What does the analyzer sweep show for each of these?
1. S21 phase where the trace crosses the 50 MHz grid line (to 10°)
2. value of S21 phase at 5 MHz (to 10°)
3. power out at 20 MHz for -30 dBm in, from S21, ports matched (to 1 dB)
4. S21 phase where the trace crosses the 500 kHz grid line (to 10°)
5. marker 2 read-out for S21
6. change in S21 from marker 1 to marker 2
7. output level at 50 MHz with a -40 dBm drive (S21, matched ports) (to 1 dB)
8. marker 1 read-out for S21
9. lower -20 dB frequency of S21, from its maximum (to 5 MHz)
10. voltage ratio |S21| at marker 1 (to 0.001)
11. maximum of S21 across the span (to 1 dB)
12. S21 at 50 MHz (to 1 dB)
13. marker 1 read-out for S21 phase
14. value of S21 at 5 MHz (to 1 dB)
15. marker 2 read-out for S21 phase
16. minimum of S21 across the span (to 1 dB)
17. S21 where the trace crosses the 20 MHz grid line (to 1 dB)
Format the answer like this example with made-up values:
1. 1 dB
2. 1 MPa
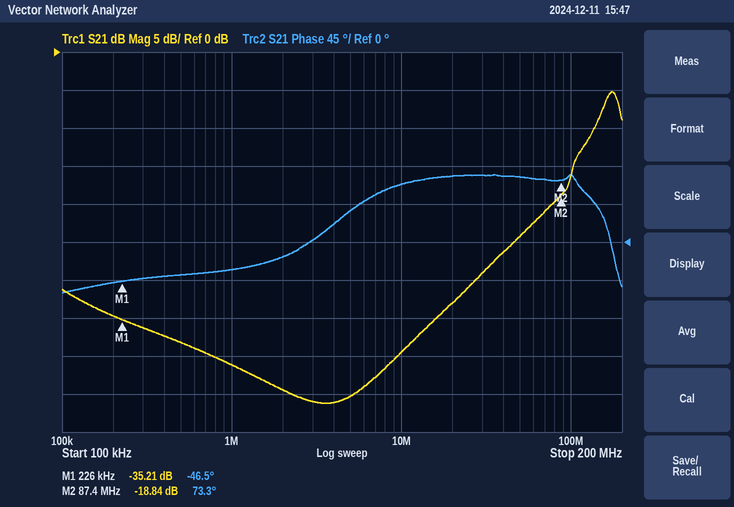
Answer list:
1. 80°
2. 40°
3. -63 dBm
4. -40°
5. -18.84 dB
6. 16.37 dB
7. -64 dBm
8. -35.21 dB
9. 45 MHz
10. 0.017
11. -5 dB
12. -24 dB
13. -46.5°
14. -45 dB
15. 73.3°
16. -46 dB
17. -33 dB
